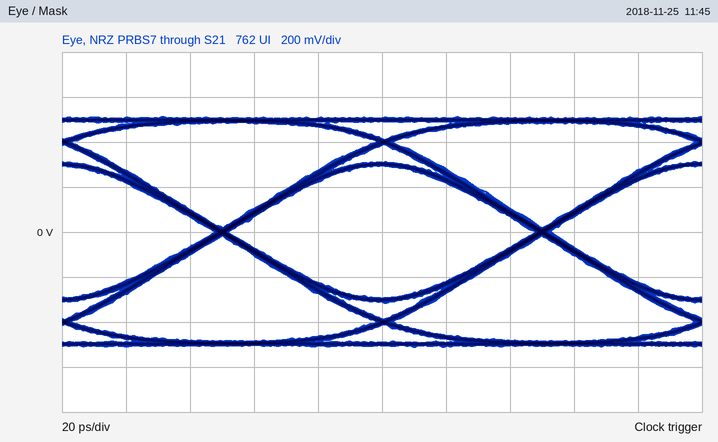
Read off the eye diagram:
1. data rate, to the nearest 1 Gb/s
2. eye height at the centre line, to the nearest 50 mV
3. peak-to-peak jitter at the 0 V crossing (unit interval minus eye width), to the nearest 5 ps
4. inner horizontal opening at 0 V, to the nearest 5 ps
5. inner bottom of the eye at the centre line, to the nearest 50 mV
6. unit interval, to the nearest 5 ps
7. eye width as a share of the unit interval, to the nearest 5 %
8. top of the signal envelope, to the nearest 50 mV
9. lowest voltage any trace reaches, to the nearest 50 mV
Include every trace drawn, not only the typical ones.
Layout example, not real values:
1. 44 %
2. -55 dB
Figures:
1. 10 Gb/s
2. 600 mV
3. 5 ps
4. 95 ps
5. -300 mV
6. 100 ps
7. 95 %
8. 500 mV
9. -500 mV
